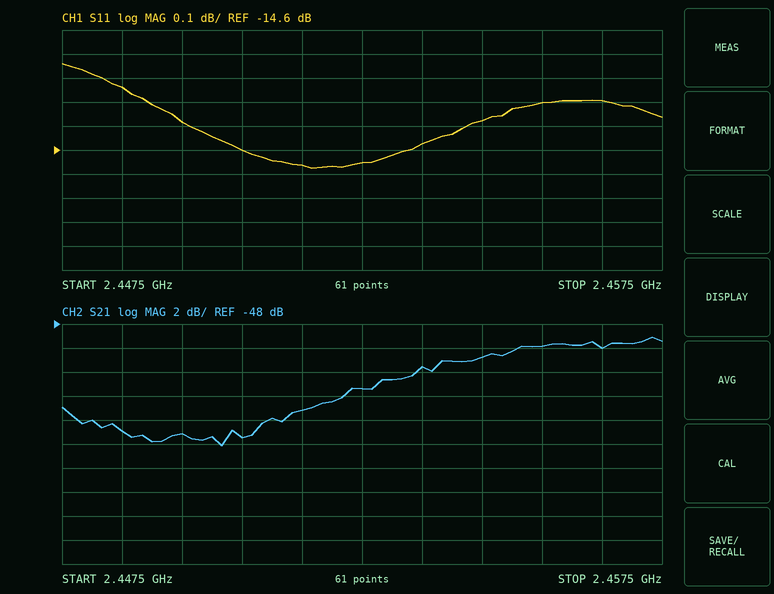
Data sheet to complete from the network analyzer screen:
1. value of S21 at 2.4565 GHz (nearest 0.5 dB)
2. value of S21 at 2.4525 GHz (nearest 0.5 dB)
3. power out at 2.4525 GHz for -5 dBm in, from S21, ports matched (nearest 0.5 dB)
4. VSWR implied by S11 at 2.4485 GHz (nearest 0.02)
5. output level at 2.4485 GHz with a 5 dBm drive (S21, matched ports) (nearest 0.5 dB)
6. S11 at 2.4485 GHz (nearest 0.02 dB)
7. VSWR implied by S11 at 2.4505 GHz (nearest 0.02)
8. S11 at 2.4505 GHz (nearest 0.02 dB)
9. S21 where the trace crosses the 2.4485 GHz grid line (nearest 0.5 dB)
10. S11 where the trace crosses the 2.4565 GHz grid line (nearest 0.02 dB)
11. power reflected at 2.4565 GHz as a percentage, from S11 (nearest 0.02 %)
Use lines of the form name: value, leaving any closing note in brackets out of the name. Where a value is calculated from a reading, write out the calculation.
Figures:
value of S21 at 2.4565 GHz: -50.0 dB
value of S21 at 2.4525 GHz: -53.5 dB
power out at 2.4525 GHz for -5 dBm in, from S21, ports matched: -5 dBm + (-53.5 dB) = -58.5 dBm
VSWR implied by S11 at 2.4485 GHz: |Γ| = 10^(-14.34/20) = 0.1919; VSWR = (1 + 0.1919)/(1 − 0.1919) ≈ 1.47, so 1.48 to the nearest 0.02
output level at 2.4485 GHz with a 5 dBm drive (S21, matched ports): 5 dBm + (-57.0 dB) = -52.0 dBm
S11 at 2.4485 GHz: -14.34 dB
VSWR implied by S11 at 2.4505 GHz: |Γ| = 10^(-14.6/20) = 0.1862; VSWR = (1 + 0.1862)/(1 − 0.1862) ≈ 1.46
S11 at 2.4505 GHz: -14.60 dB
S21 where the trace crosses the 2.4485 GHz grid line: -57.0 dB
S11 where the trace crosses the 2.4565 GHz grid line: -14.40 dB
power reflected at 2.4565 GHz as a percentage, from S11: 10^(-14.4/10) ≈ 3.63 %, so 3.64 % to the nearest 0.02 %
